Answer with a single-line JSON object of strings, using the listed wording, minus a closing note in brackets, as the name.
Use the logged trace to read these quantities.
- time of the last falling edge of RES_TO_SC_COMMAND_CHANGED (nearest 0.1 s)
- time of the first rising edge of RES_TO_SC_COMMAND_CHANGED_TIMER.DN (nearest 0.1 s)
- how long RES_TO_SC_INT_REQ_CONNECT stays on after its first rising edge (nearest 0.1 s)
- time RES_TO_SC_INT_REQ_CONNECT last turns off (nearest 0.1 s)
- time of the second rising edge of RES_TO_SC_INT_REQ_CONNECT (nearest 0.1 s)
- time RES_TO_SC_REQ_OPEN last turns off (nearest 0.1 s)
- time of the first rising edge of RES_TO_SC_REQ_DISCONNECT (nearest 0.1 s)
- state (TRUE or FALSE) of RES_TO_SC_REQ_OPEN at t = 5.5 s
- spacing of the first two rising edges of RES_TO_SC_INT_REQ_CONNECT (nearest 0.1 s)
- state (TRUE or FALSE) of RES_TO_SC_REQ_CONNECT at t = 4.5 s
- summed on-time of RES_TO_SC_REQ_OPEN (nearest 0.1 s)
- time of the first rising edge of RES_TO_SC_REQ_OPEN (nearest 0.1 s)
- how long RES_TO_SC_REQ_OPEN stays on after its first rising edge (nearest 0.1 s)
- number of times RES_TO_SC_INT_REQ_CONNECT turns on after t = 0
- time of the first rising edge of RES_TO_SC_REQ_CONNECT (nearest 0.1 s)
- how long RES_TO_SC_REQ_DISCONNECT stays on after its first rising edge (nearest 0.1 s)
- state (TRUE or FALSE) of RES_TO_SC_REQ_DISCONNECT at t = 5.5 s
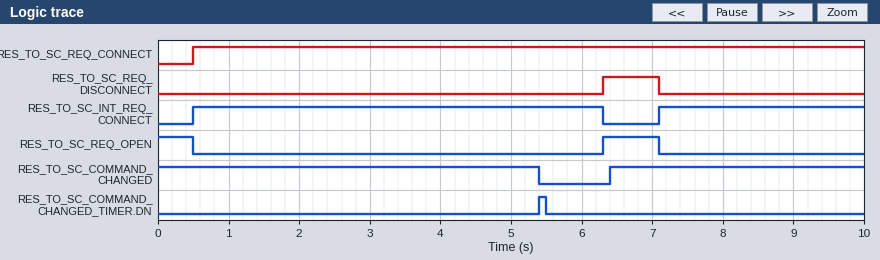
{"time of the last falling edge of RES_TO_SC_COMMAND_CHANGED": "5.4 s", "time of the first rising edge of RES_TO_SC_COMMAND_CHANGED_TIMER.DN": "5.4 s", "how long RES_TO_SC_INT_REQ_CONNECT stays on after its first rising edge": "5.8 s", "time RES_TO_SC_INT_REQ_CONNECT last turns off": "6.3 s", "time of the second rising edge of RES_TO_SC_INT_REQ_CONNECT": "7.1 s", "time RES_TO_SC_REQ_OPEN last turns off": "7.1 s", "time of the first rising edge of RES_TO_SC_REQ_DISCONNECT": "6.3 s", "state (TRUE or FALSE) of RES_TO_SC_REQ_OPEN at t = 5.5 s": "FALSE", "spacing of the first two rising edges of RES_TO_SC_INT_REQ_CONNECT": "6.6 s", "state (TRUE or FALSE) of RES_TO_SC_REQ_CONNECT at t = 4.5 s": "TRUE", "summed on-time of RES_TO_SC_REQ_OPEN": "1.3 s", "time of the first rising edge of RES_TO_SC_REQ_OPEN": "6.3 s", "how long RES_TO_SC_REQ_OPEN stays on after its first rising edge": "0.8 s", "number of times RES_TO_SC_INT_REQ_CONNECT turns on after t = 0": "2", "time of the first rising edge of RES_TO_SC_REQ_CONNECT": "0.5 s", "how long RES_TO_SC_REQ_DISCONNECT stays on after its first rising edge": "0.8 s", "state (TRUE or FALSE) of RES_TO_SC_REQ_DISCONNECT at t = 5.5 s": "FALSE"}
